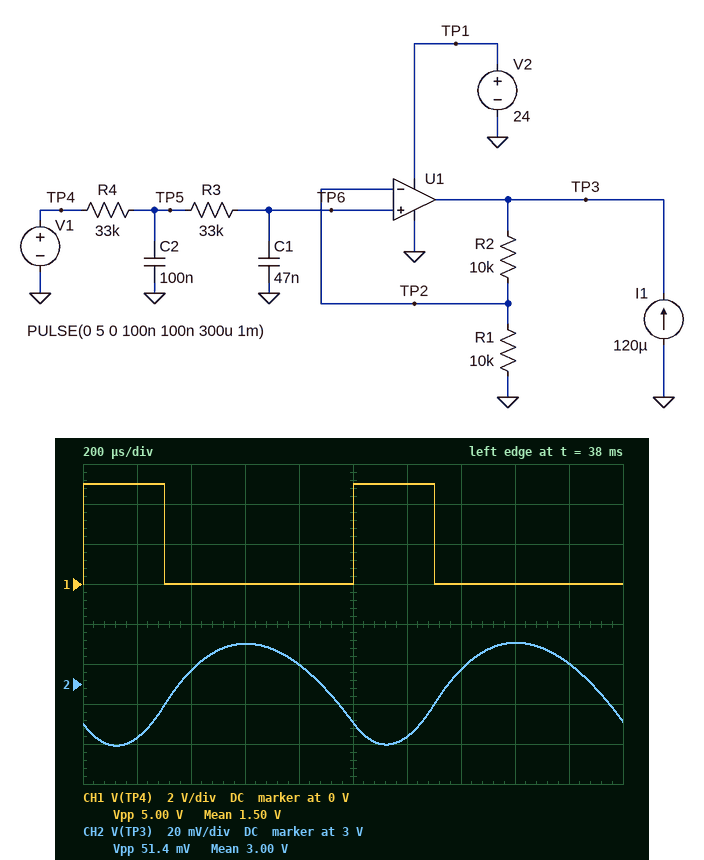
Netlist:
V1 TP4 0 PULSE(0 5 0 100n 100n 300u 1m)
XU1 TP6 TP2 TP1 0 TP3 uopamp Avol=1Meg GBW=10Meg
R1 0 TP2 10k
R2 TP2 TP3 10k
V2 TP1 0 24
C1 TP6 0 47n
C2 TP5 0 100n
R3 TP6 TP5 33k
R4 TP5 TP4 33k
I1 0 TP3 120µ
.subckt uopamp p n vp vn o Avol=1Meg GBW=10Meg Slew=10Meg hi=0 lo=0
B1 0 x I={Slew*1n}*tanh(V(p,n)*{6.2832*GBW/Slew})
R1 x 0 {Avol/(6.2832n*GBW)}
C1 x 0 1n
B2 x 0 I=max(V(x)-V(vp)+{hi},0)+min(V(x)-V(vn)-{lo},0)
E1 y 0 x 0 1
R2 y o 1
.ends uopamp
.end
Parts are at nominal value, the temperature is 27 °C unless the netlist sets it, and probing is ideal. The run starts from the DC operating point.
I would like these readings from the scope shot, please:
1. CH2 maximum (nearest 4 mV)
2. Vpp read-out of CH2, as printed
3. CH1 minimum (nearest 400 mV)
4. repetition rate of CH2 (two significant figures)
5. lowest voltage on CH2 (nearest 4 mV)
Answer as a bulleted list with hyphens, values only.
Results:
- 3.020 V
- 51.4 mV
- 0 V
- 1.0 kHz
- 2.968 V
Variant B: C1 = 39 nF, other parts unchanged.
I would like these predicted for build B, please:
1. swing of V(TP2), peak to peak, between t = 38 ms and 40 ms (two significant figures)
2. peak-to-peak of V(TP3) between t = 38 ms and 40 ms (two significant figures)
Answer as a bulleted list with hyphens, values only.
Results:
- 31 mV
- 61 mV
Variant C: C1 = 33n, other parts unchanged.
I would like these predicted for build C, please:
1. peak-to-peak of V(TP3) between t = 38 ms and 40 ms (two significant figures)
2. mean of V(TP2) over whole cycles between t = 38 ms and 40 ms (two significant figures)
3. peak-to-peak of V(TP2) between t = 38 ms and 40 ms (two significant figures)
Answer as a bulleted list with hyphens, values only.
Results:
- 72 mV
- 1.5 V
- 36 mV
